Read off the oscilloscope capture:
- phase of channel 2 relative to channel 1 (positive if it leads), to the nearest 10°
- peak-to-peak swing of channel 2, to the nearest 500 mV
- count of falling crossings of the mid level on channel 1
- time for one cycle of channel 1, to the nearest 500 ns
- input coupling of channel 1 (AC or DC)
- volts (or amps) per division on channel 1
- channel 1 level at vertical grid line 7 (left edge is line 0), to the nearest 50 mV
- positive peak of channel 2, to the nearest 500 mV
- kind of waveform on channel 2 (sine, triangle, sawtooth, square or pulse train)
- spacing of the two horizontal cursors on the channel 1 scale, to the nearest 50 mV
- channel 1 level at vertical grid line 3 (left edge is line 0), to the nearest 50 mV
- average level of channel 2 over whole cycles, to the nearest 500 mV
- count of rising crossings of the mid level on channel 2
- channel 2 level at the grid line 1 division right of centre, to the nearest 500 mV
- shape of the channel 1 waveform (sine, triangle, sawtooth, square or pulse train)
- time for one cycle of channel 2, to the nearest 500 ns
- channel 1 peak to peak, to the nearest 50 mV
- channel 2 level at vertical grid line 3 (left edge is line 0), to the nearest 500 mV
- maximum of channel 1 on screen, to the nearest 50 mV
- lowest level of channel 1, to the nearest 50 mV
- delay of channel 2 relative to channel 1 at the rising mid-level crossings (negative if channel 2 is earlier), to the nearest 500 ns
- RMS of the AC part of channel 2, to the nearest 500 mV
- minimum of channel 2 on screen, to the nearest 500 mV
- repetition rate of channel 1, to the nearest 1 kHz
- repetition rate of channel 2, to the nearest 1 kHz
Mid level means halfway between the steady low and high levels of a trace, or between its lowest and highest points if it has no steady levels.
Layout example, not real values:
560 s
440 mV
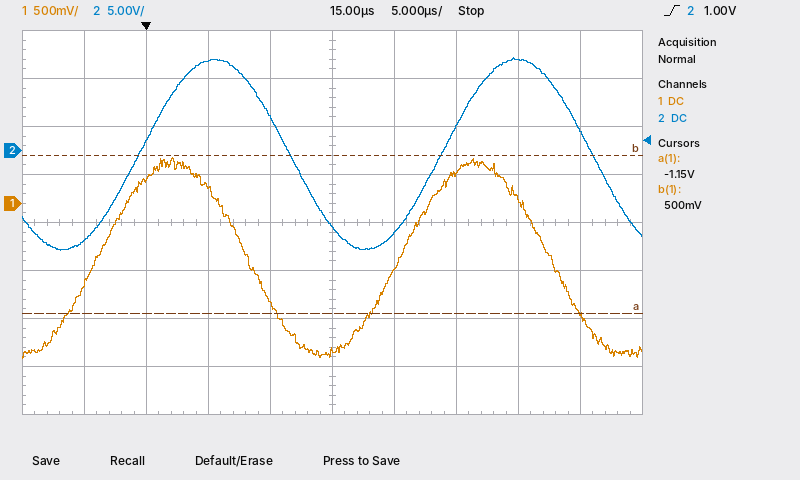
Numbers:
-50°
20.0 V
2
24.5 µs
DC
500 mV
300 mV
9.5 V
sine
1.65 V
150 mV
-500 mV
2
-8.5 V
sine
24.5 µs
2.10 V
9.5 V
500 mV
-1.60 V
+3.5 µs
7.0 V
-10.5 V
41 kHz
41 kHz
